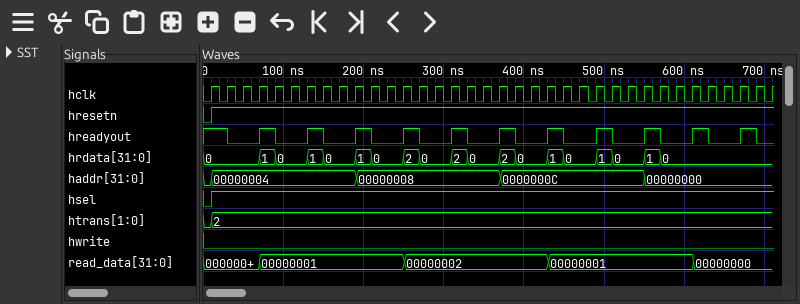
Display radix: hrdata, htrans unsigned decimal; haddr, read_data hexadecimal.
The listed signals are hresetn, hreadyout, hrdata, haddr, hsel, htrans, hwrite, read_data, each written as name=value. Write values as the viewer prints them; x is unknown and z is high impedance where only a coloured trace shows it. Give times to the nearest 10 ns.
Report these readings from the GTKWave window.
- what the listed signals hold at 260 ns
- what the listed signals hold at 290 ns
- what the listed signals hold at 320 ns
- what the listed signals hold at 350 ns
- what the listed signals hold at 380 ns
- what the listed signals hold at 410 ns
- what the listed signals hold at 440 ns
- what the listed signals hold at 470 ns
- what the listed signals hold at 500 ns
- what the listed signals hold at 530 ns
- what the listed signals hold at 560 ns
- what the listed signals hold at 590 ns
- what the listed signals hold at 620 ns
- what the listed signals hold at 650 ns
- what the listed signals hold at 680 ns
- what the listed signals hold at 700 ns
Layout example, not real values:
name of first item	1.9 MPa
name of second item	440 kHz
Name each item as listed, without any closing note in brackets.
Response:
what the listed signals hold at 260 ns	hresetn=1, hreadyout=1, hrdata=2, haddr=00000008, hsel=1, htrans=2, hwrite=0, read_data=00000002
what the listed signals hold at 290 ns	hresetn=1, hreadyout=0, hrdata=0, haddr=00000008, hsel=1, htrans=2, hwrite=0, read_data=00000002
what the listed signals hold at 320 ns	hresetn=1, hreadyout=1, hrdata=2, haddr=00000008, hsel=1, htrans=2, hwrite=0, read_data=00000002
what the listed signals hold at 350 ns	hresetn=1, hreadyout=0, hrdata=0, haddr=00000008, hsel=1, htrans=2, hwrite=0, read_data=00000002
what the listed signals hold at 380 ns	hresetn=1, hreadyout=1, hrdata=2, haddr=0000000C, hsel=1, htrans=2, hwrite=0, read_data=00000002
what the listed signals hold at 410 ns	hresetn=1, hreadyout=0, hrdata=0, haddr=0000000C, hsel=1, htrans=2, hwrite=0, read_data=00000002
what the listed signals hold at 440 ns	hresetn=1, hreadyout=1, hrdata=1, haddr=0000000C, hsel=1, htrans=2, hwrite=0, read_data=00000001
what the listed signals hold at 470 ns	hresetn=1, hreadyout=0, hrdata=0, haddr=0000000C, hsel=1, htrans=2, hwrite=0, read_data=00000001
what the listed signals hold at 500 ns	hresetn=1, hreadyout=1, hrdata=1, haddr=0000000C, hsel=1, htrans=2, hwrite=0, read_data=00000001
what the listed signals hold at 530 ns	hresetn=1, hreadyout=0, hrdata=0, haddr=0000000C, hsel=1, htrans=2, hwrite=0, read_data=00000001
what the listed signals hold at 560 ns	hresetn=1, hreadyout=1, hrdata=1, haddr=00000000, hsel=1, htrans=2, hwrite=0, read_data=00000001
what the listed signals hold at 590 ns	hresetn=1, hreadyout=0, hrdata=0, haddr=00000000, hsel=1, htrans=2, hwrite=0, read_data=00000001
what the listed signals hold at 620 ns	hresetn=1, hreadyout=1, hrdata=0, haddr=00000000, hsel=1, htrans=2, hwrite=0, read_data=00000000
what the listed signals hold at 650 ns	hresetn=1, hreadyout=0, hrdata=0, haddr=00000000, hsel=1, htrans=2, hwrite=0, read_data=00000000
what the listed signals hold at 680 ns	hresetn=1, hreadyout=1, hrdata=0, haddr=00000000, hsel=1, htrans=2, hwrite=0, read_data=00000000
what the listed signals hold at 700 ns	hresetn=1, hreadyout=0, hrdata=0, haddr=00000000, hsel=1, htrans=2, hwrite=0, read_data=00000000
